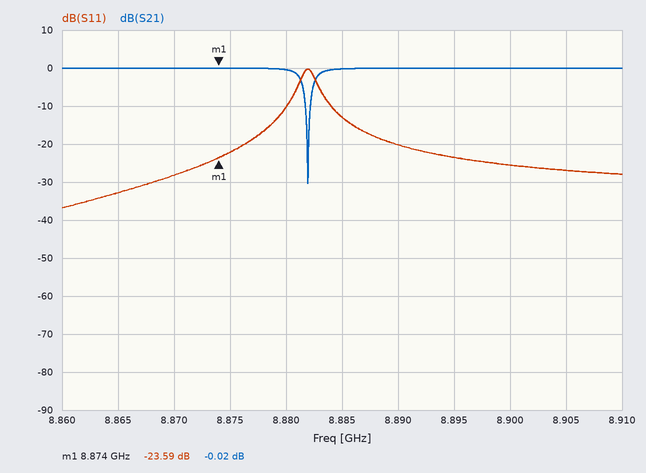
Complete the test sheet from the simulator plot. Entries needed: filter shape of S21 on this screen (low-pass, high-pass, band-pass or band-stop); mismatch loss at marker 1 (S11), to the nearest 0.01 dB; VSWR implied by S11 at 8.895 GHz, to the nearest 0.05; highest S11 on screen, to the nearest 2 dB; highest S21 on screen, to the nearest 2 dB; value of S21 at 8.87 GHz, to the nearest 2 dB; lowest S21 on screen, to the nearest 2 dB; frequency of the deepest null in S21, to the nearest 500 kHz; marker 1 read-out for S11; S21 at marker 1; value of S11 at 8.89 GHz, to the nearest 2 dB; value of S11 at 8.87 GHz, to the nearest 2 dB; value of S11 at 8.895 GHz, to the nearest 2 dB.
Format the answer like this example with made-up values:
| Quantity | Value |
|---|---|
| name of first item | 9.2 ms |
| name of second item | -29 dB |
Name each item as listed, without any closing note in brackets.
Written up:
| Quantity | Value |
|---|---|
| filter shape of S21 on this screen | band-stop |
| mismatch loss at marker 1 (S11), to the nearest 0.01 dB | 0.02 dB |
| VSWR implied by S11 at 8.895 GHz, to the nearest 0.05 | 1.15 |
| highest S11 on screen, to the nearest 2 dB | 0 dB |
| highest S21 on screen, to the nearest 2 dB | 0 dB |
| value of S21 at 8.87 GHz, to the nearest 2 dB | 0 dB |
| lowest S21 on screen, to the nearest 2 dB | -30 dB |
| frequency of the deepest null in S21, to the nearest 500 kHz | 8.8820 GHz |
| marker 1 read-out for S11 | -23.59 dB |
| S21 at marker 1 | -0.02 dB |
| value of S11 at 8.89 GHz, to the nearest 2 dB | -20 dB |
| value of S11 at 8.87 GHz, to the nearest 2 dB | -28 dB |
| value of S11 at 8.895 GHz, to the nearest 2 dB | -24 dB |
